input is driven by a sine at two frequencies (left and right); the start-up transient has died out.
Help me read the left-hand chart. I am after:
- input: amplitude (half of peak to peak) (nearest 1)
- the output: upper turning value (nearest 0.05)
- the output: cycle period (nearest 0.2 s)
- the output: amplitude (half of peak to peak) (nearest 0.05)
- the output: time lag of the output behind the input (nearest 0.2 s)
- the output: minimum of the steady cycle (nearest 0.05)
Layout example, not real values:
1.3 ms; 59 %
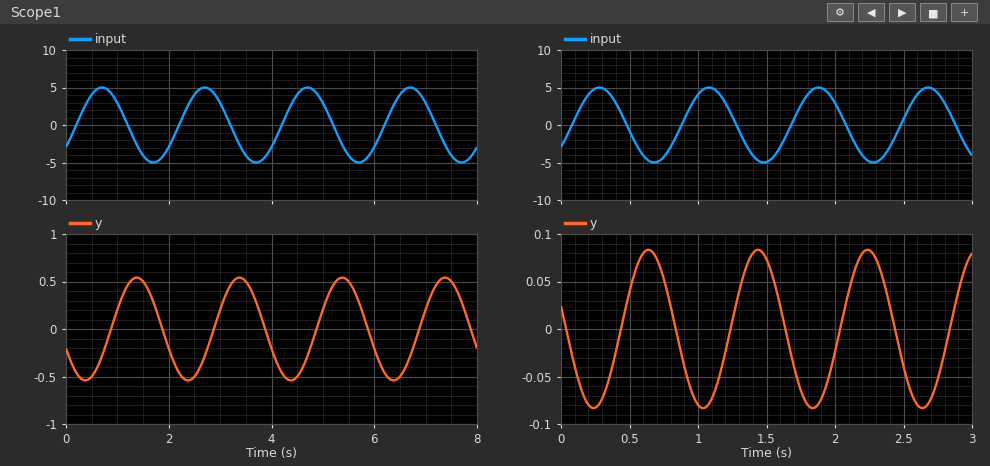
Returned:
5; 0.55; 2.0 s; 0.55; 0.6 s; -0.55
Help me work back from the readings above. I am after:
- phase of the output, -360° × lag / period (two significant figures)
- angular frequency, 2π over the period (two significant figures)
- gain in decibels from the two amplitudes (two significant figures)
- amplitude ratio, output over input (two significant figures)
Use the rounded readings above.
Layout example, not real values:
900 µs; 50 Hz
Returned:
-110°; 3.1 rad/s; -19 dB; 0.11
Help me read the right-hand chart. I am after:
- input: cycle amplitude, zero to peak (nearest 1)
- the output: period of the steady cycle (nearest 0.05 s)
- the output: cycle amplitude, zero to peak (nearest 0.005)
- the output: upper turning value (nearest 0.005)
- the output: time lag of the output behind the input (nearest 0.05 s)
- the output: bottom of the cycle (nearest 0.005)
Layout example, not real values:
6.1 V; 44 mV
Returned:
5; 0.80 s; 0.085; 0.085; 0.35 s; -0.085
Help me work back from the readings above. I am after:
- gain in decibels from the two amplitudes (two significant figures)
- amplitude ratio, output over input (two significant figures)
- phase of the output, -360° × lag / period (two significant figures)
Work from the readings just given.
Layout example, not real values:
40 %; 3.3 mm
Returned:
-35 dB; 0.017; -160°
